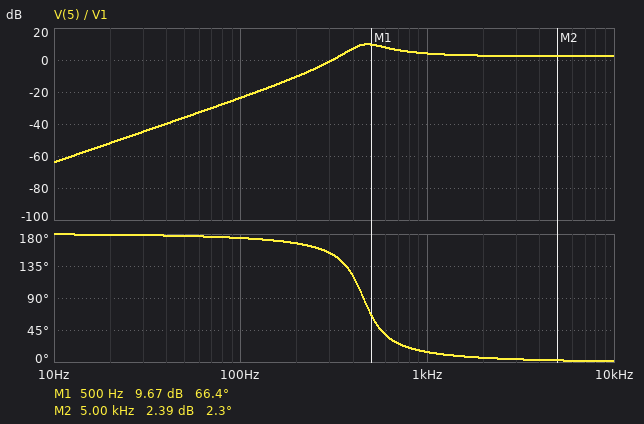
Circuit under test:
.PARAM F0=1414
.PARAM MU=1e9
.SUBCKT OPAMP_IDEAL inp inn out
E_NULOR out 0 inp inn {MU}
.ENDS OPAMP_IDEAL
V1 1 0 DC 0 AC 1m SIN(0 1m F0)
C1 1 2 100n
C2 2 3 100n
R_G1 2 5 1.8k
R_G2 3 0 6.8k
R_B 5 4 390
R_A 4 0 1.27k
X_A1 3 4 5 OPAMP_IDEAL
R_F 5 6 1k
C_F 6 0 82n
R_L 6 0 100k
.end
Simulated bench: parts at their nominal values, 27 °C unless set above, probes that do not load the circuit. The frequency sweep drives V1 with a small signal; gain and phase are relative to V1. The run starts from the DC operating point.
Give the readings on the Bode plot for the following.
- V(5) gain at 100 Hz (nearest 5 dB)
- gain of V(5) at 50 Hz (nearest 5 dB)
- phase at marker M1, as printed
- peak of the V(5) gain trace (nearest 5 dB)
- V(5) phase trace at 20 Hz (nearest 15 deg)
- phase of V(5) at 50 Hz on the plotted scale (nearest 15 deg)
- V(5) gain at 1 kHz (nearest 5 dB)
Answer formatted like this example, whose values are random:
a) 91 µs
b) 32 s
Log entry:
a) -25 dB
b) -35 dB
c) 66.4 deg
d) 10 dB
e) 180 deg
f) 180 deg
g) 5 dB
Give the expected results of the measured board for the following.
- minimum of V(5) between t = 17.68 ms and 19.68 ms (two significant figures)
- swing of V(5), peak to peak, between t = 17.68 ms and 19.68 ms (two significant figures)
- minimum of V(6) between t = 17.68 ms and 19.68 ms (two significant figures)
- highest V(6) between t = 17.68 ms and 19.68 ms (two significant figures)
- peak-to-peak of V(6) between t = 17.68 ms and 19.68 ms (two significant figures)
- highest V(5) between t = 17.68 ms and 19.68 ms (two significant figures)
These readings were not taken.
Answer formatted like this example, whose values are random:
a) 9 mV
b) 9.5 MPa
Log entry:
a) -1.4 mV
b) 2.9 mV
c) -1.2 mV
d) 1.2 mV
e) 2.3 mV
f) 1.4 mV
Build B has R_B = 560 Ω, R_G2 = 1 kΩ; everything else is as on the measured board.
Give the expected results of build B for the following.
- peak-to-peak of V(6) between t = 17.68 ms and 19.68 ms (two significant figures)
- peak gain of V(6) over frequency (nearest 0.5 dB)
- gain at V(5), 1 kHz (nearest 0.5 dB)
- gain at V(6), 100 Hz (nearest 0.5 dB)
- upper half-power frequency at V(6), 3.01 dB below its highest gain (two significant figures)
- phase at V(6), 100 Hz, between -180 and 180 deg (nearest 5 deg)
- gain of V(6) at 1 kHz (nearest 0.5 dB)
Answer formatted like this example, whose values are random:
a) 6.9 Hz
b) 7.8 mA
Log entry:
a) 1.2 mV
b) -3.5 dB
c) -6.0 dB
d) -40.0 dB
e) 5.2 kHz
f) 165 deg
g) -7.0 dB
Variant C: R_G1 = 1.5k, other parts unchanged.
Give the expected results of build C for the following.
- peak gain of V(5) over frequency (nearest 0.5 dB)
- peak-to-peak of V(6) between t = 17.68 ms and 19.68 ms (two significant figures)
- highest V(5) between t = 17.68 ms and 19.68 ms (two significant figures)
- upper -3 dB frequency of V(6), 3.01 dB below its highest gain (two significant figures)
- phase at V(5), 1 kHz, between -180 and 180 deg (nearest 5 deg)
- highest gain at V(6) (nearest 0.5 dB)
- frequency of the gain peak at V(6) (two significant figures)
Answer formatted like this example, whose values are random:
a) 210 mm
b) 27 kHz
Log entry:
a) 13.5 dB
b) 2.4 mV
c) 1.5 mV
d) 600 Hz
e) 10 deg
f) 13.0 dB
g) 510 Hz
